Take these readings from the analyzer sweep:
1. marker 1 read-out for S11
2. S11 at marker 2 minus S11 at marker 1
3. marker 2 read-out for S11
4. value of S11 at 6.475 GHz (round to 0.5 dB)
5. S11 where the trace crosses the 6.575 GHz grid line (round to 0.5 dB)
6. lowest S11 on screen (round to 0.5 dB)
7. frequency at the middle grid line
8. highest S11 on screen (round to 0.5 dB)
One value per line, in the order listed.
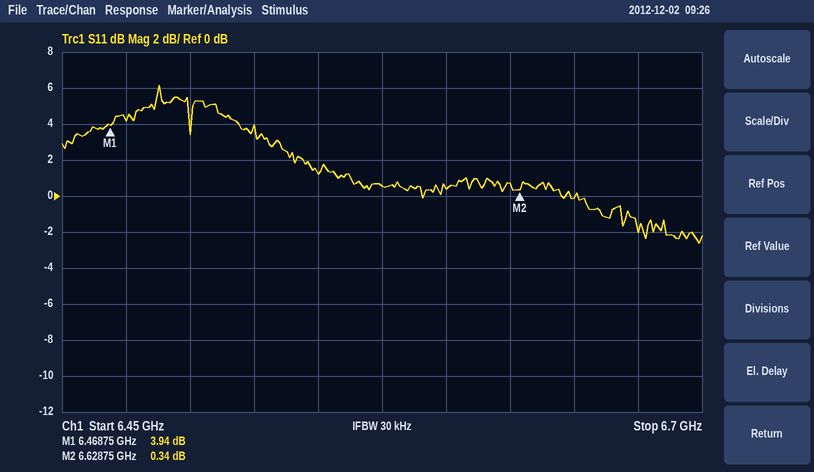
3.94 dB
-3.60 dB
0.34 dB
4.0 dB
0.5 dB
-2.5 dB
6.575 GHz
6.0 dB
